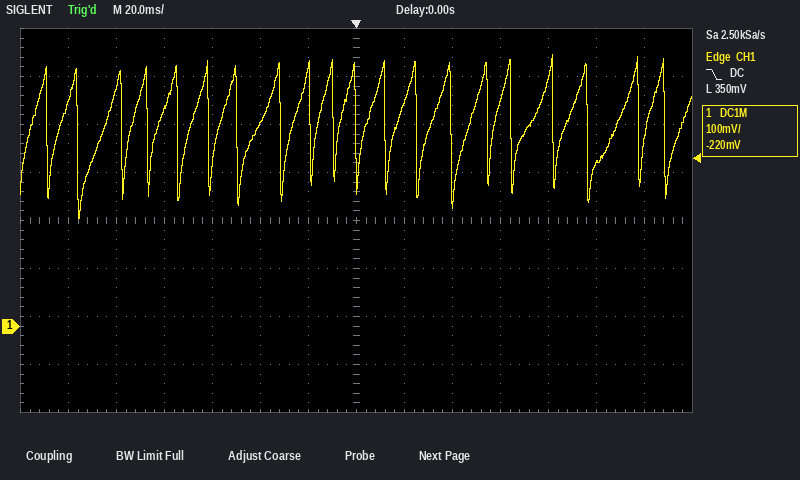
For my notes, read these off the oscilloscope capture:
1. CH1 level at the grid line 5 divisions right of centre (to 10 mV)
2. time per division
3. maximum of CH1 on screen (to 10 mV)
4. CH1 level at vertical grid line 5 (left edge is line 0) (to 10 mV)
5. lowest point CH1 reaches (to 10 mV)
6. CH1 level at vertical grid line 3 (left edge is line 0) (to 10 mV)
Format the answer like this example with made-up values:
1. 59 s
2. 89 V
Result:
1. 340 mV
2. 20 ms
3. 570 mV
4. 420 mV
5. 220 mV
6. 450 mV
